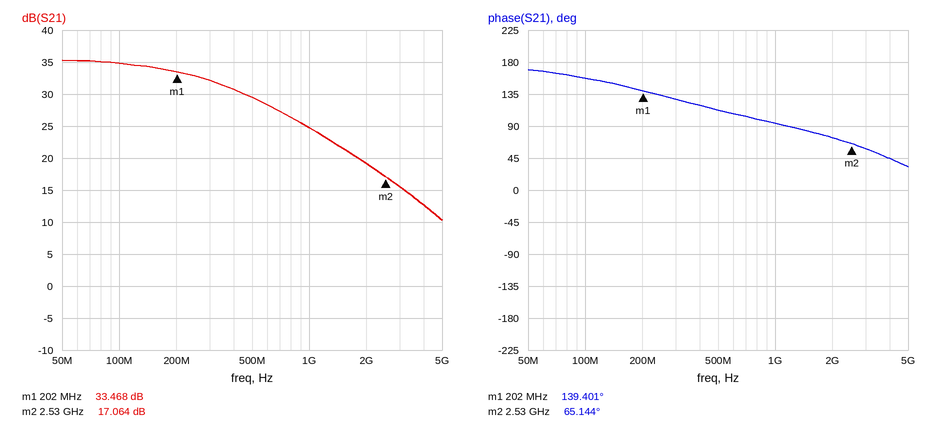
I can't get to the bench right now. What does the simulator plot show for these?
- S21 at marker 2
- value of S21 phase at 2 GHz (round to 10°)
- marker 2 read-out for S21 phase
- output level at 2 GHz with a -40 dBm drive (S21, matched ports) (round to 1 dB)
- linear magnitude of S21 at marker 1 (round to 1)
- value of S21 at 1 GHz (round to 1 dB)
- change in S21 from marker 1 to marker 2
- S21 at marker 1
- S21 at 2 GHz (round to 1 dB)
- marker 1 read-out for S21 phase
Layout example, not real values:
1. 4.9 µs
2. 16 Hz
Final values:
1. 17.064 dB
2. 70°
3. 65.144°
4. -21 dBm
5. 47
6. 25 dB
7. -16.404 dB
8. 33.468 dB
9. 19 dB
10. 139.401°
